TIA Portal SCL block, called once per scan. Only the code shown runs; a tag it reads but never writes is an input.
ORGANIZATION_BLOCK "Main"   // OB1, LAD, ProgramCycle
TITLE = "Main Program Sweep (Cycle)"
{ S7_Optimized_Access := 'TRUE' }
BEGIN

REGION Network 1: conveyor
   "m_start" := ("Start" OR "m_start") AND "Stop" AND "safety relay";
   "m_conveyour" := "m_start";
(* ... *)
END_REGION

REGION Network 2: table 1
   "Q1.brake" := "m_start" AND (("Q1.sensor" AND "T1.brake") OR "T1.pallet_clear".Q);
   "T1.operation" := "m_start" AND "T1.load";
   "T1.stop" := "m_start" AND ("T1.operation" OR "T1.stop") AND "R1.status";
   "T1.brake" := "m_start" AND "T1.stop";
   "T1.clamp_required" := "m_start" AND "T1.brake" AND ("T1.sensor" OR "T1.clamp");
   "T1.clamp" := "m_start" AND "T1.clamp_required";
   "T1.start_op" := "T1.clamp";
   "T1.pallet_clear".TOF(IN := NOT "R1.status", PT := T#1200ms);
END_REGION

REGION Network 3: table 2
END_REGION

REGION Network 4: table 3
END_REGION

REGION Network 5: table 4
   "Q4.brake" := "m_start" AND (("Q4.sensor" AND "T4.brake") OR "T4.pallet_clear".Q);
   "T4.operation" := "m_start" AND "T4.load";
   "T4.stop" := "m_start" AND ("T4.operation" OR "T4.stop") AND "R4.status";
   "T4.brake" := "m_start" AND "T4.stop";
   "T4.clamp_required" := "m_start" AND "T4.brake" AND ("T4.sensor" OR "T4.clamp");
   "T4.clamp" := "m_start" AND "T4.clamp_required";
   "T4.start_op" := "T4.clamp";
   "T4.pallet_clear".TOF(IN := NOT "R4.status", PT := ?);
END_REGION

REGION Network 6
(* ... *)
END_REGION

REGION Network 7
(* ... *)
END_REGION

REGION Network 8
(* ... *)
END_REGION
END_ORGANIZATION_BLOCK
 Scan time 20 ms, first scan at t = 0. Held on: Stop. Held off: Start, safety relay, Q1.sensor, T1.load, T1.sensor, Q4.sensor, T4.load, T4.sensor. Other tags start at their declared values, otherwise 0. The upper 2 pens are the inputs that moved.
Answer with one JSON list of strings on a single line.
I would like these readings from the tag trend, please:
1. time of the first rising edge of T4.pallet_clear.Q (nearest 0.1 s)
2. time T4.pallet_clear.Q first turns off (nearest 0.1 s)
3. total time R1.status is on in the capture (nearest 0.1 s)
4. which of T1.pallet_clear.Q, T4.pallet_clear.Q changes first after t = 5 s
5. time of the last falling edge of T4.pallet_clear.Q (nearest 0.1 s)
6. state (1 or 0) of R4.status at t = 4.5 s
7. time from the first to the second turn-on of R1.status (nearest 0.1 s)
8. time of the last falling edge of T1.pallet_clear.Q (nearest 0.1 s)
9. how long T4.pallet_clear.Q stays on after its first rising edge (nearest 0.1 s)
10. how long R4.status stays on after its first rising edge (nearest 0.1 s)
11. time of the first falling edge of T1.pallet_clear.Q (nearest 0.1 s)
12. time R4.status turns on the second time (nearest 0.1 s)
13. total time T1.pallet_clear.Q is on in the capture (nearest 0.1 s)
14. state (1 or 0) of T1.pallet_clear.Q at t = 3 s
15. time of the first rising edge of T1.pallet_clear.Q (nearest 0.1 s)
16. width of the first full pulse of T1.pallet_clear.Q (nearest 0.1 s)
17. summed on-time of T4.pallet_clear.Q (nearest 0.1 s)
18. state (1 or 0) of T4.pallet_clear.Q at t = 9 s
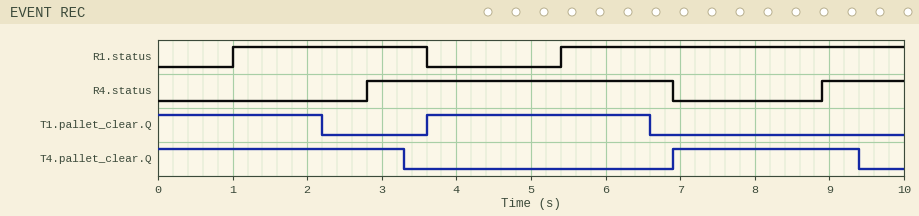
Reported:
["6.9 s", "3.3 s", "7.2 s", "T1.pallet_clear.Q", "9.4 s", "1", "4.4 s", "6.6 s", "2.5 s", "4.1 s", "2.2 s", "8.9 s", "5.2 s", "0", "3.6 s", "3.0 s", "5.8 s", "1"]
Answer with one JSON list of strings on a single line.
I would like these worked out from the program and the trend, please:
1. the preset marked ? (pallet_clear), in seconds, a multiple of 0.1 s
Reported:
["0.5 s"]
